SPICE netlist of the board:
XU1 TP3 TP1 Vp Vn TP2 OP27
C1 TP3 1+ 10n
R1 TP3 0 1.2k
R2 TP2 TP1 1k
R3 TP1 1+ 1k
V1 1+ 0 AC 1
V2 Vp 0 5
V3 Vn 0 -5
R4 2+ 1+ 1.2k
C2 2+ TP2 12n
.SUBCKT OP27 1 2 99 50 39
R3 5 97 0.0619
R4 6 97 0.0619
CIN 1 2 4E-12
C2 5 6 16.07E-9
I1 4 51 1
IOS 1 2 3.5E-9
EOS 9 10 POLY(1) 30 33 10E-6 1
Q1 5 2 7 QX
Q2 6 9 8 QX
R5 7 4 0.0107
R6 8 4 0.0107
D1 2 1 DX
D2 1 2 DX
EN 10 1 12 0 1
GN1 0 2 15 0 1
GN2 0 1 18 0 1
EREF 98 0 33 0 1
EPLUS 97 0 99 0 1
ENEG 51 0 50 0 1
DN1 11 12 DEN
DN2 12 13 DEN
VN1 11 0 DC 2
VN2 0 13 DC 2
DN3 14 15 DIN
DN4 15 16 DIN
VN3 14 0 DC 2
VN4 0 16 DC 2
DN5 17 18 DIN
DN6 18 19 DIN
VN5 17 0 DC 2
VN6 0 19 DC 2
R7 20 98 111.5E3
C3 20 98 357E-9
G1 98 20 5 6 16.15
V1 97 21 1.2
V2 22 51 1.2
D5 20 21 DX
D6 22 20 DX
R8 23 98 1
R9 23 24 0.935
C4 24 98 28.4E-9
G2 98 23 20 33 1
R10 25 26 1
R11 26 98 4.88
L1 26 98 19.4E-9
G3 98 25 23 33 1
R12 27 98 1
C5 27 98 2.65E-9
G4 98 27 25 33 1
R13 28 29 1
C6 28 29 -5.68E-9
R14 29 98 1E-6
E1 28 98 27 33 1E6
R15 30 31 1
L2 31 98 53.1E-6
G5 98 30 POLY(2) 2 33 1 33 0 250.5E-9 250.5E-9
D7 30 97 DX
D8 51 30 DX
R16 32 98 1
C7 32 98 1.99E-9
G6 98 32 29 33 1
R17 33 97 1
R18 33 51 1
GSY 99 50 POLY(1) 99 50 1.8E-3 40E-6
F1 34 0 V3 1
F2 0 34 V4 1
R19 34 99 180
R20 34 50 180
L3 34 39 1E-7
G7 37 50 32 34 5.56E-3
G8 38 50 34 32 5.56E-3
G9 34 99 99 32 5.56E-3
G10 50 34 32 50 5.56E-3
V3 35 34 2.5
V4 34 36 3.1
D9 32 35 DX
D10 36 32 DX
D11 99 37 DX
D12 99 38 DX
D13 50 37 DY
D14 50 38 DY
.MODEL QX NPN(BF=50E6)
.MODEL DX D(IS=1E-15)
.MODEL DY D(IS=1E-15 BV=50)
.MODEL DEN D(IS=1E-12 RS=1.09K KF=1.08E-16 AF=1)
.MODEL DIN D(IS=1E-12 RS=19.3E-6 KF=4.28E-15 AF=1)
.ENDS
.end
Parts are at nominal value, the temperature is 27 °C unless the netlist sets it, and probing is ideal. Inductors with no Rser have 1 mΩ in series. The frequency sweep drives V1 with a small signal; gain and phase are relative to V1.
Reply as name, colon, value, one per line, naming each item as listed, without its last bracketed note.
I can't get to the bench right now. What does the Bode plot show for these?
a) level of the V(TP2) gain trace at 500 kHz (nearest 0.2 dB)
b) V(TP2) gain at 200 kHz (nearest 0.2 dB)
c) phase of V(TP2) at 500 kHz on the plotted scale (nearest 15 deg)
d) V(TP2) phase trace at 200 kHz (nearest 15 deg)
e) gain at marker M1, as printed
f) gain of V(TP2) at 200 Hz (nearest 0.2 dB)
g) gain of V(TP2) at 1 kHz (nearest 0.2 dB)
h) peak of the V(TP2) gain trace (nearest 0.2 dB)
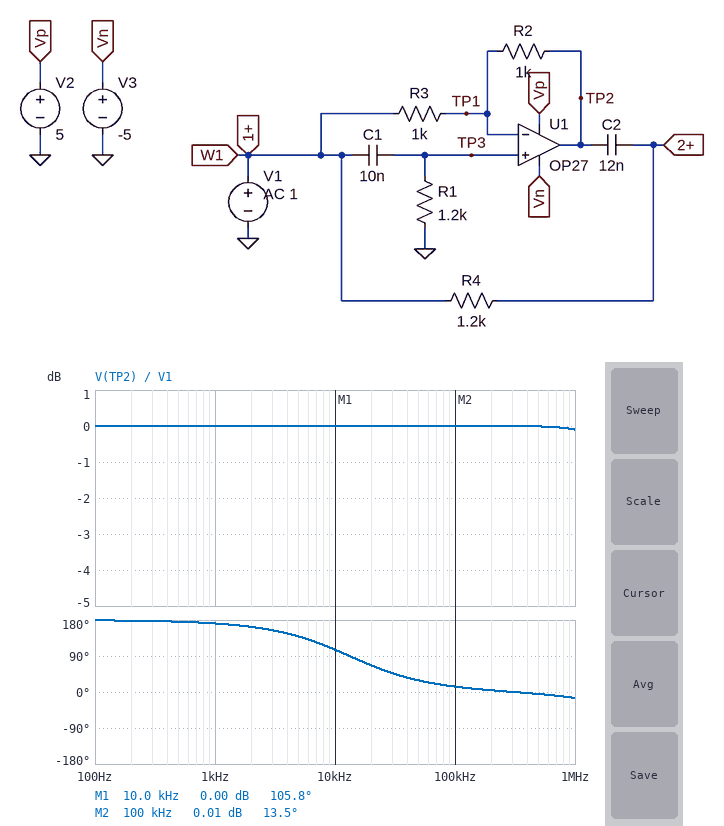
level of the V(TP2) gain trace at 500 kHz: 0 dB
V(TP2) gain at 200 kHz: 0 dB
phase of V(TP2) at 500 kHz on the plotted scale: 0 deg
V(TP2) phase trace at 200 kHz: 0 deg
gain at marker M1, as printed: 0.00 dB
gain of V(TP2) at 200 Hz: 0 dB
gain of V(TP2) at 1 kHz: 0 dB
peak of the V(TP2) gain trace: 0 dB
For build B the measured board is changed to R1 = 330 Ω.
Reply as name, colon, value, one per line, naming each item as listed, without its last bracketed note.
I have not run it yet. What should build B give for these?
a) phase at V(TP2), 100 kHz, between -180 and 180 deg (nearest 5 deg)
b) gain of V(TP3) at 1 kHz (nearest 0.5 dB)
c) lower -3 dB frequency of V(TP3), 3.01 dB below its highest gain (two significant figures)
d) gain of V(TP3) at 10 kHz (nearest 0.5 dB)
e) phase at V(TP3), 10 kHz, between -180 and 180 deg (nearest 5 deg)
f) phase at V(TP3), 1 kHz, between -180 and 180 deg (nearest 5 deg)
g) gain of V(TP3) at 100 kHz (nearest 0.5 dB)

phase at V(TP2), 100 kHz, between -180 and 180 deg: 50 deg
gain of V(TP3) at 1 kHz: -33.5 dB
lower -3 dB frequency of V(TP3), 3.01 dB below its highest gain: 48 kHz
gain of V(TP3) at 10 kHz: -14.0 dB
phase at V(TP3), 10 kHz, between -180 and 180 deg: 80 deg
phase at V(TP3), 1 kHz, between -180 and 180 deg: 90 deg
gain of V(TP3) at 100 kHz: -1.0 dB
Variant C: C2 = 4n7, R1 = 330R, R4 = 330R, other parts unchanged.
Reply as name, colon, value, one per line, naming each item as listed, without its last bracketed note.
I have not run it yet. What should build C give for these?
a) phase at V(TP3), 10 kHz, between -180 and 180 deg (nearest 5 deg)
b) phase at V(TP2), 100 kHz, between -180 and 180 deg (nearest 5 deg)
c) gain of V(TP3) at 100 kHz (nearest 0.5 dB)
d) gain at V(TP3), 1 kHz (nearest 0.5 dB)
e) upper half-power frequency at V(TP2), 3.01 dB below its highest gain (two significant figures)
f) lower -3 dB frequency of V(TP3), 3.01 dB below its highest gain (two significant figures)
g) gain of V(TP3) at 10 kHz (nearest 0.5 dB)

phase at V(TP3), 10 kHz, between -180 and 180 deg: 80 deg
phase at V(TP2), 100 kHz, between -180 and 180 deg: 50 deg
gain of V(TP3) at 100 kHz: -1.0 dB
gain at V(TP3), 1 kHz: -33.5 dB
upper half-power frequency at V(TP2), 3.01 dB below its highest gain: 2.8 MHz
lower -3 dB frequency of V(TP3), 3.01 dB below its highest gain: 48 kHz
gain of V(TP3) at 10 kHz: -14.0 dB
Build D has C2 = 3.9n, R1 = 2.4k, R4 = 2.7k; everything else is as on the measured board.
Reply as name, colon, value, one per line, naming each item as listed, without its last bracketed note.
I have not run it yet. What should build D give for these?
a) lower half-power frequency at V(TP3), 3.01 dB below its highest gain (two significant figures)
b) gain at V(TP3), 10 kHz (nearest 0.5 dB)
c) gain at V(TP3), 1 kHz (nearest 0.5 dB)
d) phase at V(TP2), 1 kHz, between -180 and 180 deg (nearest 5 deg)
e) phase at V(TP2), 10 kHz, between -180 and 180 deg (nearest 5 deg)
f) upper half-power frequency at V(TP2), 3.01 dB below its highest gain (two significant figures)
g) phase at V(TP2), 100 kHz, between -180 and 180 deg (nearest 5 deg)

lower half-power frequency at V(TP3), 3.01 dB below its highest gain: 6.6 kHz
gain at V(TP3), 10 kHz: -1.5 dB
gain at V(TP3), 1 kHz: -16.5 dB
phase at V(TP2), 1 kHz, between -180 and 180 deg: 165 deg
phase at V(TP2), 10 kHz, between -180 and 180 deg: 65 deg
upper half-power frequency at V(TP2), 3.01 dB below its highest gain: 3.5 MHz
phase at V(TP2), 100 kHz, between -180 and 180 deg: 5 deg
